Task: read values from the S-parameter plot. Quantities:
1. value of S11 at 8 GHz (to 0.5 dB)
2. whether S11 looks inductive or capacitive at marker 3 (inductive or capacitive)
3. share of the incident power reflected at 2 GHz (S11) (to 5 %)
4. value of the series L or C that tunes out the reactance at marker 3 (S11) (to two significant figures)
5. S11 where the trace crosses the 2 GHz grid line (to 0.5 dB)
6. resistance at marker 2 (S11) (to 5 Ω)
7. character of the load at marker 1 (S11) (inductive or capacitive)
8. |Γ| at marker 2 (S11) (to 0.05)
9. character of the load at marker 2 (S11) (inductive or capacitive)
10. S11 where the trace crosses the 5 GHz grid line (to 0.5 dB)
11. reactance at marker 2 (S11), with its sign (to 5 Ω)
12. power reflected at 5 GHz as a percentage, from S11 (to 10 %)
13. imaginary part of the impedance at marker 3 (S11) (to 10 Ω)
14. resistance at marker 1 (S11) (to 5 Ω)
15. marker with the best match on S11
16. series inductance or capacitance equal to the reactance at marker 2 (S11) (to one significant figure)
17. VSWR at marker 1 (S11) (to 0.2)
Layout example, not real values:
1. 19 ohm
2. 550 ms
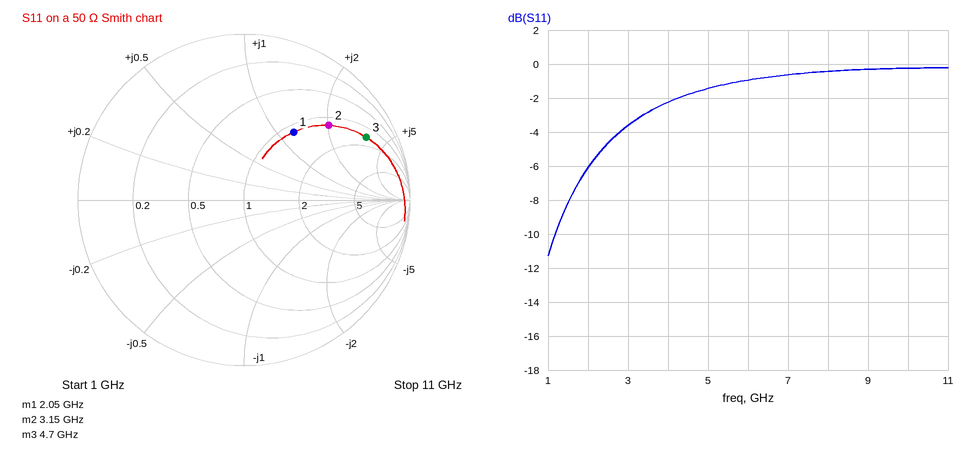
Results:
1. -0.5 dB
2. inductive
3. 25 %
4. 190 fF
5. -6.0 dB
6. 60 Ω
7. inductive
8. 0.70
9. inductive
10. -1.5 dB
11. +100 Ω
12. 70 %
13. +180 Ω
14. 55 Ω
15. marker 1
16. 5 nH
17. 3.0
